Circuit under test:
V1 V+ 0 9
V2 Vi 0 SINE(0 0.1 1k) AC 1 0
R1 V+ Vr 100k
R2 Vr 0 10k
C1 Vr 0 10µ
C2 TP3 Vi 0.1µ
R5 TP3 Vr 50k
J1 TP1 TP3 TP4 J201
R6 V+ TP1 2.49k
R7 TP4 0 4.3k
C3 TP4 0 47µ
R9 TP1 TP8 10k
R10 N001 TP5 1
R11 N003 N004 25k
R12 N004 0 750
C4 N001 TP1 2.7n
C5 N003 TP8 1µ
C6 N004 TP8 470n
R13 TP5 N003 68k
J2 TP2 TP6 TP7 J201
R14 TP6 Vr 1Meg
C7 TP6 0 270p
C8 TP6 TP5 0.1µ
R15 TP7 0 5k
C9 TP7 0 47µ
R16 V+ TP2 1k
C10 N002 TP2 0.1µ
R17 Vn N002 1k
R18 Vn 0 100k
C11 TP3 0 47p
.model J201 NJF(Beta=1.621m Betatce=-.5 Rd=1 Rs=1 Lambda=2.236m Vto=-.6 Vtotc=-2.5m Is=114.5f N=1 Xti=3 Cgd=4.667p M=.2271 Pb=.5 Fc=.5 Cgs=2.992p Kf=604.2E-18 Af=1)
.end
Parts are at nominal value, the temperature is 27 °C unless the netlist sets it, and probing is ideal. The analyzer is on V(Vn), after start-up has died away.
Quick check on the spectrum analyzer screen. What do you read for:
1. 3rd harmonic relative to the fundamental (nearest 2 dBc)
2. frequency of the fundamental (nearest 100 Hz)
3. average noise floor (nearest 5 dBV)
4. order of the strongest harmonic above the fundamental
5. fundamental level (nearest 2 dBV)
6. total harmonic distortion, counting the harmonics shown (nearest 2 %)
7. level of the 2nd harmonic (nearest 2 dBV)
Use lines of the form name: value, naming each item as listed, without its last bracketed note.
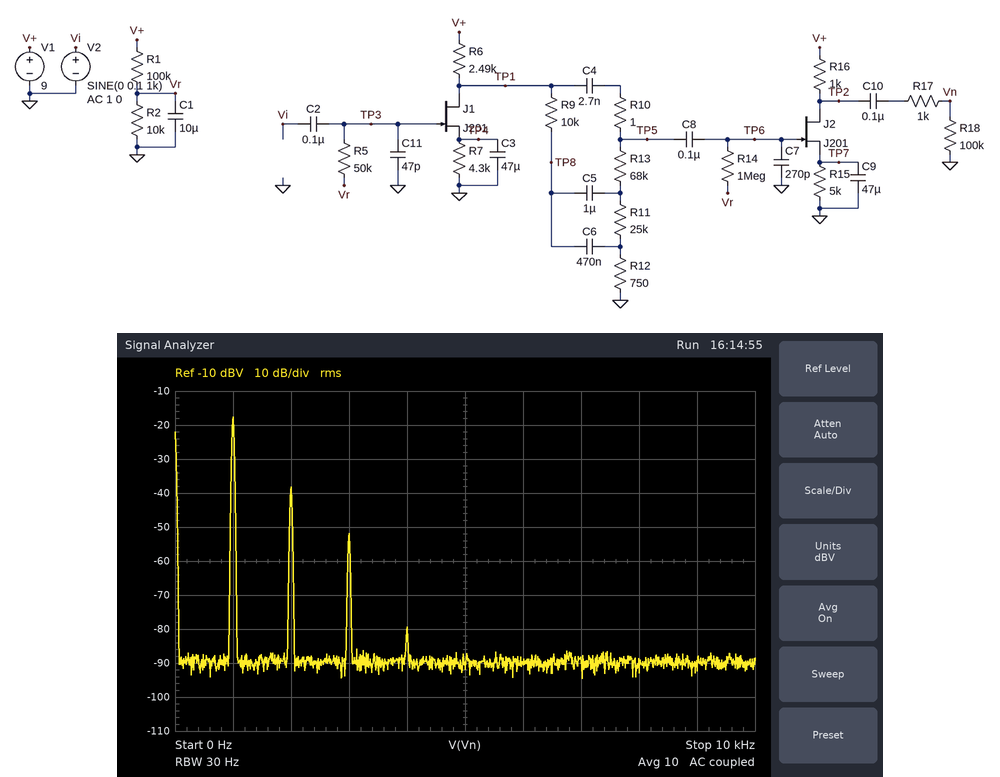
3rd harmonic relative to the fundamental: -34 dBc
frequency of the fundamental: 1.0 kHz
average noise floor: -90 dBV
order of the strongest harmonic above the fundamental: 2
fundamental level: -18 dBV
total harmonic distortion, counting the harmonics shown: 10 %
level of the 2nd harmonic: -38 dBV
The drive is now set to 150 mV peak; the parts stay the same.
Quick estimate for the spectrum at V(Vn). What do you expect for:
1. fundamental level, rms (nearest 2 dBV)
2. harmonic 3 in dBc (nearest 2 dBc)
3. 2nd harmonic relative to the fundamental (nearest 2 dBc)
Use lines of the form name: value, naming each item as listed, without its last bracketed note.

fundamental level, rms: -14 dBV
harmonic 3 in dBc: -26 dBc
2nd harmonic relative to the fundamental: -16 dBc
